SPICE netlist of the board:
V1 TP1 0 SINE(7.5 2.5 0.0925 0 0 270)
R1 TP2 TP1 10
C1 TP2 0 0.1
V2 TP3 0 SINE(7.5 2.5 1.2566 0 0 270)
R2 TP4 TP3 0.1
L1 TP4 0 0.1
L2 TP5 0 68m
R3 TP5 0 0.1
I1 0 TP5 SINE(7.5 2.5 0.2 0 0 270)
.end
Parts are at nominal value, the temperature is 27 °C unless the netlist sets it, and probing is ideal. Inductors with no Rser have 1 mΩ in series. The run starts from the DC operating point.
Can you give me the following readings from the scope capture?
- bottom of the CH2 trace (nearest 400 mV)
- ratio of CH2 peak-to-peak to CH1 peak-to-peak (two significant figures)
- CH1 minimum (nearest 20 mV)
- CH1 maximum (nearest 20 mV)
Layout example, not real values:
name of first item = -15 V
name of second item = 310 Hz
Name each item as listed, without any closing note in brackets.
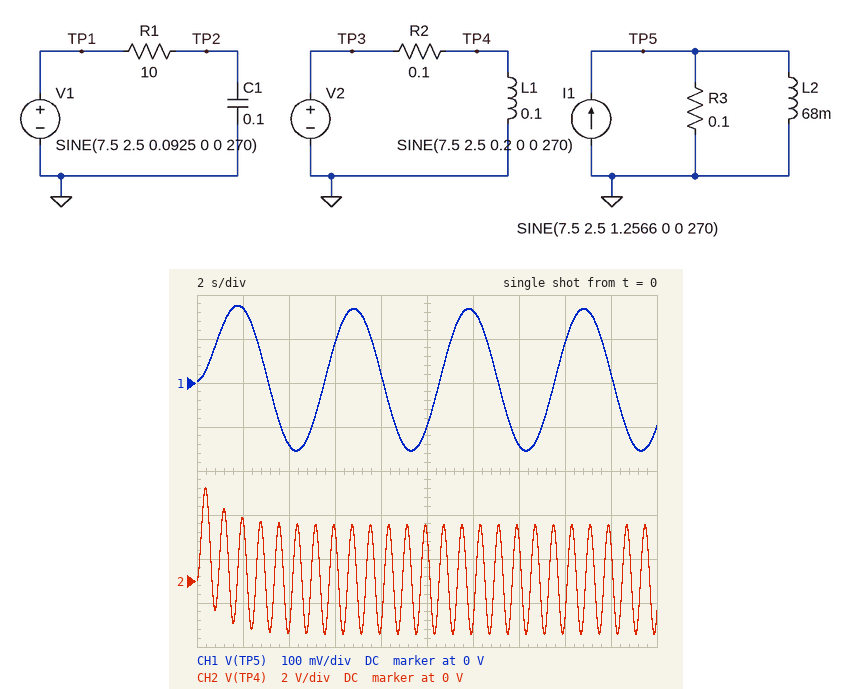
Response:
bottom of the CH2 trace = -2.4 V
ratio of CH2 peak-to-peak to CH1 peak-to-peak = 20
CH1 minimum = -160 mV
CH1 maximum = 180 mV
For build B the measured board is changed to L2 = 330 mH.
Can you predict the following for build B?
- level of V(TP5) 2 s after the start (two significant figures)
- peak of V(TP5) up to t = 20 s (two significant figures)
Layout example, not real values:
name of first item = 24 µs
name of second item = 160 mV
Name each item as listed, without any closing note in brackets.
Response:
level of V(TP5) 2 s after the start = 360 mV
peak of V(TP5) up to t = 20 s = 370 mV
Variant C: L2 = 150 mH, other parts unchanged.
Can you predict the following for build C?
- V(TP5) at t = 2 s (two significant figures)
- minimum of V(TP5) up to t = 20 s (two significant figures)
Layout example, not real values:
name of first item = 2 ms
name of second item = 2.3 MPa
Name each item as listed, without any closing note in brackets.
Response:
V(TP5) at t = 2 s = 280 mV
minimum of V(TP5) up to t = 20 s = -210 mV
